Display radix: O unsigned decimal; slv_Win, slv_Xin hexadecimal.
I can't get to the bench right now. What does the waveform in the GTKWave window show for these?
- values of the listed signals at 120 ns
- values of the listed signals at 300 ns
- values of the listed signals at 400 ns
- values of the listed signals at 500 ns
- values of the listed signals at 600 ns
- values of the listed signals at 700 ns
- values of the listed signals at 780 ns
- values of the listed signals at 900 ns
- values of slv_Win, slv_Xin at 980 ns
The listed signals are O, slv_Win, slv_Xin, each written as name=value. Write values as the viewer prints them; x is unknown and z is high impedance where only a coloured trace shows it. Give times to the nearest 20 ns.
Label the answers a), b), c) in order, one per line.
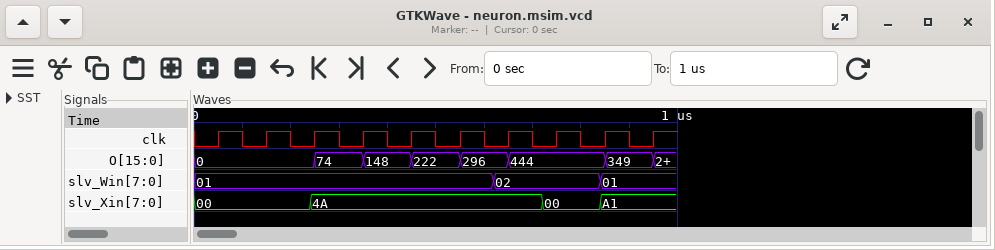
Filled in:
a) O=0, slv_Win=01, slv_Xin=00
b) O=74, slv_Win=01, slv_Xin=4A
c) O=148, slv_Win=01, slv_Xin=4A
d) O=222, slv_Win=01, slv_Xin=4A
e) O=296, slv_Win=01, slv_Xin=4A
f) O=444, slv_Win=02, slv_Xin=4A
g) O=444, slv_Win=02, slv_Xin=00
h) O=349, slv_Win=01, slv_Xin=A1
i) slv_Win=01, slv_Xin=A1
